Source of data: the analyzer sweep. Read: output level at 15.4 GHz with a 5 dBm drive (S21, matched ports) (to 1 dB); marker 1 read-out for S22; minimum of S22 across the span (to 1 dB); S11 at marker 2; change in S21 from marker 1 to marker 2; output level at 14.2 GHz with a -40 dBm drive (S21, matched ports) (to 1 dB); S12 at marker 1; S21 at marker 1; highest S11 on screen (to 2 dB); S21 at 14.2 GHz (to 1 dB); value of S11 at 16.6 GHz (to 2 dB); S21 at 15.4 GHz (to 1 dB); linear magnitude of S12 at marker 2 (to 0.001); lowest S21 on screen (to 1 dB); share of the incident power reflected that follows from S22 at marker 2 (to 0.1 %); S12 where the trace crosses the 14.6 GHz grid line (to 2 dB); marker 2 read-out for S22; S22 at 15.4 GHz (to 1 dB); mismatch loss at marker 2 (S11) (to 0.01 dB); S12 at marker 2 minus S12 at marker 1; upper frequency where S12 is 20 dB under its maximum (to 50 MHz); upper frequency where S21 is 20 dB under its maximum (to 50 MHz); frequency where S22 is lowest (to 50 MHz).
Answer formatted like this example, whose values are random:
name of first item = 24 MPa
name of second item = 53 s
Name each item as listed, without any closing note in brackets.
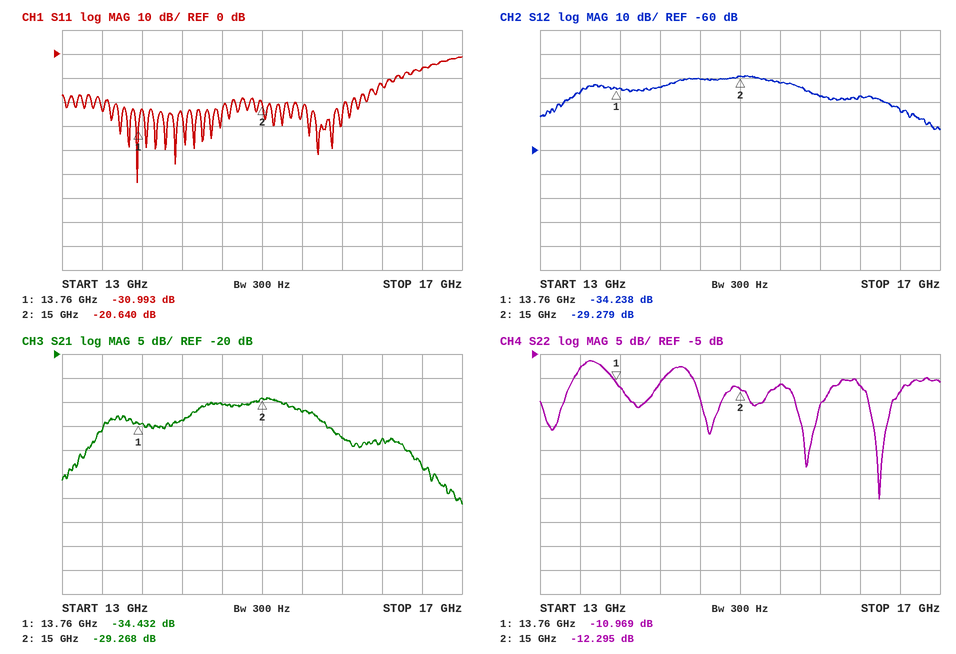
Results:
output level at 15.4 GHz with a 5 dBm drive (S21, matched ports) = -27 dBm
marker 1 read-out for S22 = -10.969 dB
minimum of S22 across the span = -35 dB
S11 at marker 2 = -20.640 dB
change in S21 from marker 1 to marker 2 = 5.164 dB
output level at 14.2 GHz with a -40 dBm drive (S21, matched ports) = -74 dBm
S12 at marker 1 = -34.238 dB
S21 at marker 1 = -34.432 dB
highest S11 on screen = -2 dB
S21 at 14.2 GHz = -34 dB
value of S11 at 16.6 GHz = -6 dB
S21 at 15.4 GHz = -32 dB
linear magnitude of S12 at marker 2 = 0.034
lowest S21 on screen = -51 dB
share of the incident power reflected that follows from S22 at marker 2 = 5.9 %
S12 where the trace crosses the 14.6 GHz grid line = -30 dB
marker 2 read-out for S22 = -12.295 dB
S22 at 15.4 GHz = -11 dB
mismatch loss at marker 2 (S11) = 0.04 dB
S12 at marker 2 minus S12 at marker 1 = 4.959 dB
upper frequency where S12 is 20 dB under its maximum = 16.85 GHz
upper frequency where S21 is 20 dB under its maximum = 16.90 GHz
frequency where S22 is lowest = 16.40 GHz
